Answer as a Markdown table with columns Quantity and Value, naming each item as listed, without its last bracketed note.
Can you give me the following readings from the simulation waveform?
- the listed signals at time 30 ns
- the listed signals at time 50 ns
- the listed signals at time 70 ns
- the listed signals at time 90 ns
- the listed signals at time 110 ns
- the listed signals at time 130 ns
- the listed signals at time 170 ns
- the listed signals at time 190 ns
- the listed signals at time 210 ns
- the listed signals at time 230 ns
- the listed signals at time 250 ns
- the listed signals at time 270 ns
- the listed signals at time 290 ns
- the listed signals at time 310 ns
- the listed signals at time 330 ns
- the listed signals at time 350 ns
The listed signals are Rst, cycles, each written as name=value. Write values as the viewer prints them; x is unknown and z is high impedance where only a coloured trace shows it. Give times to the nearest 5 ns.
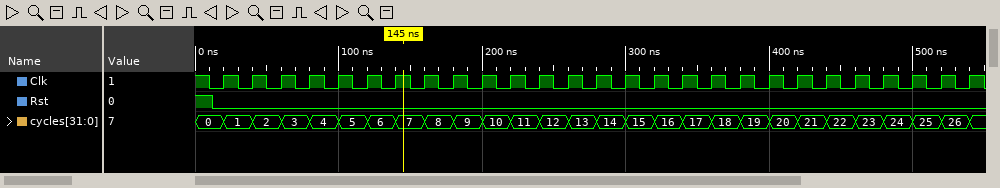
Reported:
| Quantity | Value |
|---|---|
| the listed signals at time 30 ns | Rst=0, cycles=1 |
| the listed signals at time 50 ns | Rst=0, cycles=2 |
| the listed signals at time 70 ns | Rst=0, cycles=3 |
| the listed signals at time 90 ns | Rst=0, cycles=4 |
| the listed signals at time 110 ns | Rst=0, cycles=5 |
| the listed signals at time 130 ns | Rst=0, cycles=6 |
| the listed signals at time 170 ns | Rst=0, cycles=8 |
| the listed signals at time 190 ns | Rst=0, cycles=9 |
| the listed signals at time 210 ns | Rst=0, cycles=10 |
| the listed signals at time 230 ns | Rst=0, cycles=11 |
| the listed signals at time 250 ns | Rst=0, cycles=12 |
| the listed signals at time 270 ns | Rst=0, cycles=13 |
| the listed signals at time 290 ns | Rst=0, cycles=14 |
| the listed signals at time 310 ns | Rst=0, cycles=15 |
| the listed signals at time 330 ns | Rst=0, cycles=16 |
| the listed signals at time 350 ns | Rst=0, cycles=17 |
